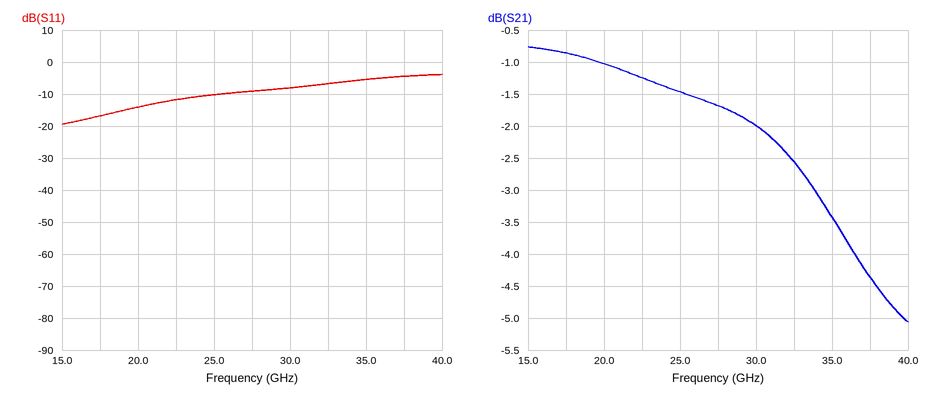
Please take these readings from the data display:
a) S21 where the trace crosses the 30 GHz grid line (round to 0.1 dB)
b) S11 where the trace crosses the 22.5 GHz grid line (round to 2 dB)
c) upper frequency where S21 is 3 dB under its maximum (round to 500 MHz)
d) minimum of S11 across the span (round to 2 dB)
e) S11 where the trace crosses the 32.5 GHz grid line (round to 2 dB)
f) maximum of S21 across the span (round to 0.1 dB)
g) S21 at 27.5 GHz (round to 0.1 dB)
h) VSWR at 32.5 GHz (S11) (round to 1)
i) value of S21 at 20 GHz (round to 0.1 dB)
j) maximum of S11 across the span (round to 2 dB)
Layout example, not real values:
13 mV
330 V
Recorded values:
-2.0 dB
-12 dB
36.0 GHz
-20 dB
-6 dB
-0.8 dB
-1.7 dB
3
-1.0 dB
-4 dB
